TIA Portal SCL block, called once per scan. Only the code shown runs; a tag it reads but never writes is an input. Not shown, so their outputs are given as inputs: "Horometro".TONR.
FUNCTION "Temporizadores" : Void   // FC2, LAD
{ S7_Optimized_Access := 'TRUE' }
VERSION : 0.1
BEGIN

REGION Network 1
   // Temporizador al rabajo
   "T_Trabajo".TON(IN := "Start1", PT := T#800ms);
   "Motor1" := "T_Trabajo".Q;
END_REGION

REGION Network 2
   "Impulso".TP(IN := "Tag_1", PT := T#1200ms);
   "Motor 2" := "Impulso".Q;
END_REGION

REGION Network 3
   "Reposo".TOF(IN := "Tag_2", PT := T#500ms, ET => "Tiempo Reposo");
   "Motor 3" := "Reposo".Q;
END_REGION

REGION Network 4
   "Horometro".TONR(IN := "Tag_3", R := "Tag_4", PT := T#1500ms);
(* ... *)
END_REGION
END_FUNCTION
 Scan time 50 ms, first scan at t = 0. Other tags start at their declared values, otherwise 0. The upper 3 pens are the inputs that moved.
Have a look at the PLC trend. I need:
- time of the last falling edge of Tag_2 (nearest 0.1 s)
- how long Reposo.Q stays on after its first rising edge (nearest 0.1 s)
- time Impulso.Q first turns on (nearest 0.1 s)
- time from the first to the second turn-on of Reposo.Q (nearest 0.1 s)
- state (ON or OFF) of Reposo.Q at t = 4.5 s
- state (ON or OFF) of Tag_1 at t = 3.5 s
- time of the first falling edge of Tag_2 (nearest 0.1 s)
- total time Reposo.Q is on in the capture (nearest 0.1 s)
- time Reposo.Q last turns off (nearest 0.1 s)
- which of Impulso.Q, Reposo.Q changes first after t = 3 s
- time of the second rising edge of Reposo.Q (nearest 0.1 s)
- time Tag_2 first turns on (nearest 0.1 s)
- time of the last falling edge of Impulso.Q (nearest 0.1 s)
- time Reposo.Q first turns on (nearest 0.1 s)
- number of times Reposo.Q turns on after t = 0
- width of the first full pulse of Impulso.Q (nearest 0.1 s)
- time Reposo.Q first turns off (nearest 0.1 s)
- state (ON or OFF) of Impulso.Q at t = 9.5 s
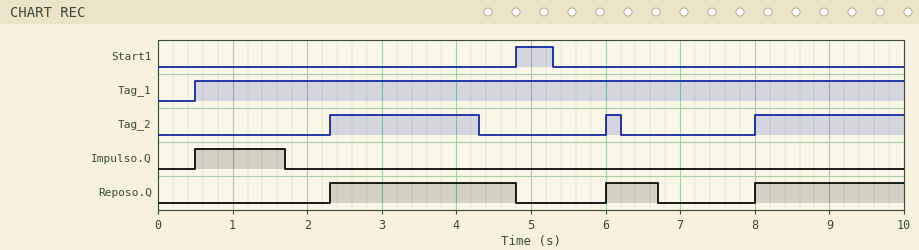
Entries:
6.2 s
2.5 s
0.5 s
3.7 s
ON
ON
4.3 s
5.2 s
6.7 s
Reposo.Q
6.0 s
2.3 s
1.7 s
2.3 s
3
1.2 s
4.8 s
OFF
